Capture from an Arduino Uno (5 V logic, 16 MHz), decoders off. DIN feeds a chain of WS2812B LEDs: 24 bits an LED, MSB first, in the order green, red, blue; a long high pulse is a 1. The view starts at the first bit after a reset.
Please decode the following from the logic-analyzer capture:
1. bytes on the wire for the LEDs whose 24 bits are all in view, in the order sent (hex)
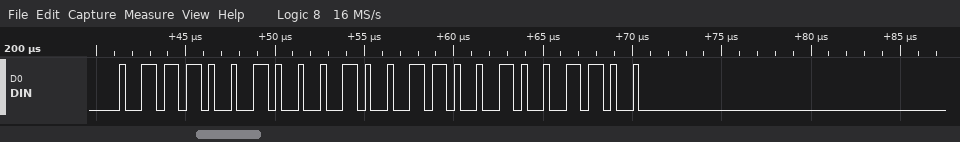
72 26 4C
